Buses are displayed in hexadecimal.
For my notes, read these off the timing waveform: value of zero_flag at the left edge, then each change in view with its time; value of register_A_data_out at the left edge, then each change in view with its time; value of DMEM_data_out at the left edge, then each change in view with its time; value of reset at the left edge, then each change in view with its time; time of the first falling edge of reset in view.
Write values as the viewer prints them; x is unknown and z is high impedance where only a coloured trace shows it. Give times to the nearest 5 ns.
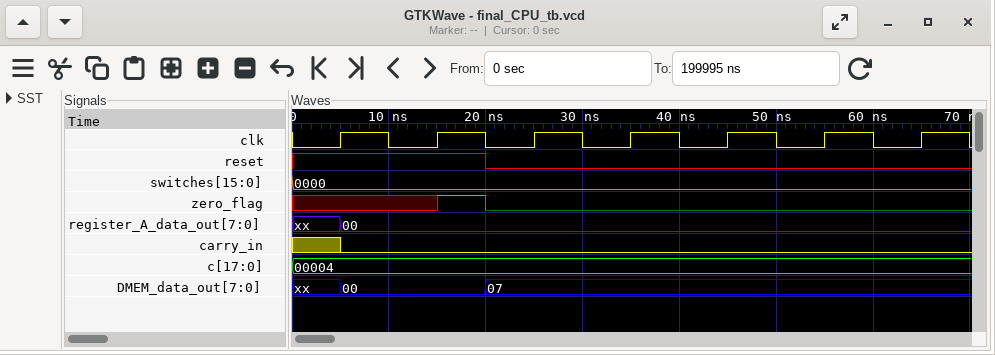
x, 1 at 15 ns, 0 at 20 ns
xx, 00 at 5 ns
xx, 00 at 5 ns, 07 at 20 ns
1, 0 at 20 ns
20 ns
